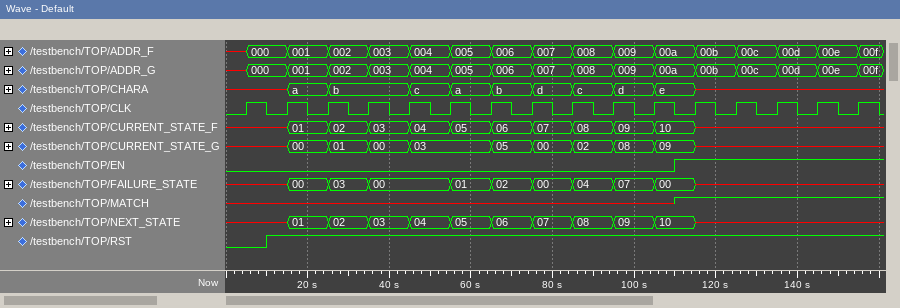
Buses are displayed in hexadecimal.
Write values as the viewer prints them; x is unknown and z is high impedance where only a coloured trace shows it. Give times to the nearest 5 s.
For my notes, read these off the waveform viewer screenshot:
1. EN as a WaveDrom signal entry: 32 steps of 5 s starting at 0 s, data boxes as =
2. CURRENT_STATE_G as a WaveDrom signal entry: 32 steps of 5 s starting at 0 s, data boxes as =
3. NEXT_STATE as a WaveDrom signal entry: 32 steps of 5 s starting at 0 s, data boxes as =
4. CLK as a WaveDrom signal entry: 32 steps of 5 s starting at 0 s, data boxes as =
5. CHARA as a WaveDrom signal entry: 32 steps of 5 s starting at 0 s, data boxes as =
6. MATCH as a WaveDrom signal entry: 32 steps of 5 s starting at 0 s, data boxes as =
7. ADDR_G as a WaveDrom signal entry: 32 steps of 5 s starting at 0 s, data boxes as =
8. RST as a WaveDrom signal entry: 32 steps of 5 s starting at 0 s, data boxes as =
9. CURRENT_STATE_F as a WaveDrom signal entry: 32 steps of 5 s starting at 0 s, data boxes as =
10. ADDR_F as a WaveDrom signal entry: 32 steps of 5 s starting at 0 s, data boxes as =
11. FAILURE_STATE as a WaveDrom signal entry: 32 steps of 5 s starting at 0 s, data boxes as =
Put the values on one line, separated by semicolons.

{name: 'EN', wave: '0.....................1.........'}; {name: 'CURRENT_STATE_G', wave: 'x..=.=.=.=...=.=.=.=.=.x........', data: '00 01 00 03 05 00 02 08 09'}; {name: 'NEXT_STATE', wave: 'x..=.=.=.=.=.=.=.=.=.=.x........', data: '01 02 03 04 05 06 07 08 09 10'}; {name: 'CLK', wave: '01010101010101010101010101010101'}; {name: 'CHARA', wave: 'x..=.=...=.=.=.=.=.=.=.x........', data: 'a b c a b d c d e'}; {name: 'MATCH', wave: 'x.....................1.........'}; {name: 'ADDR_G', wave: 'x=.=.=.=.=.=.=.=.=.=.=.=.=.=.=.=', data: '000 001 002 003 004 005 006 007 008 009 00a 00b 00c 00d 00e 00f'}; {name: 'RST', wave: '0.1.............................'}; {name: 'CURRENT_STATE_F', wave: 'x..=.=.=.=.=.=.=.=.=.=.x........', data: '01 02 03 04 05 06 07 08 09 10'}; {name: 'ADDR_F', wave: 'x=.=.=.=.=.=.=.=.=.=.=.=.=.=.=.=', data: '000 001 002 003 004 005 006 007 008 009 00a 00b 00c 00d 00e 00f'}; {name: 'FAILURE_STATE', wave: 'x..=.=.=...=.=.=.=.=.=.x........', data: '00 03 00 01 02 00 04 07 00'}
